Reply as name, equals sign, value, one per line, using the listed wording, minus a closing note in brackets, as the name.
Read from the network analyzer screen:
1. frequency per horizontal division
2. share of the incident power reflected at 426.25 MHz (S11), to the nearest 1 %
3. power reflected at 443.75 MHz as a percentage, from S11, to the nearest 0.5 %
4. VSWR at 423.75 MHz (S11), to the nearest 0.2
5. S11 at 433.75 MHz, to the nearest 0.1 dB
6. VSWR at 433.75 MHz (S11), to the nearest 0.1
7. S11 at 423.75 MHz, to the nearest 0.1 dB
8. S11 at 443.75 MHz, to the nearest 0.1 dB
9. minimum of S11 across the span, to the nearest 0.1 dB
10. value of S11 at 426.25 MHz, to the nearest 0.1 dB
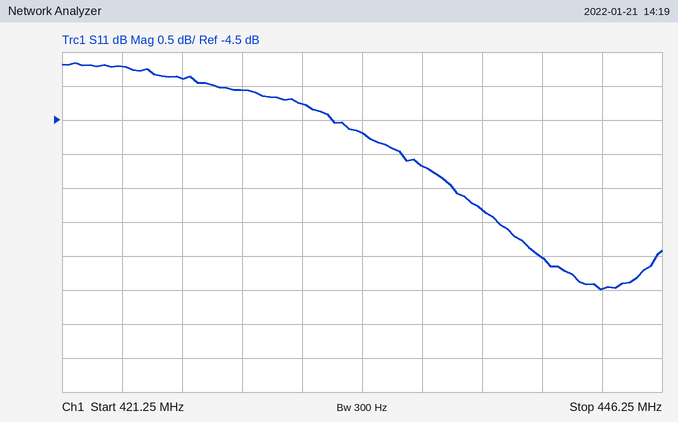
frequency per horizontal division = 2.5 MHz
share of the incident power reflected at 426.25 MHz (S11), to the nearest 1 % = 41 %
power reflected at 443.75 MHz as a percentage, from S11, to the nearest 0.5 % = 20.0 %
VSWR at 423.75 MHz (S11), to the nearest 0.2 = 4.8
S11 at 433.75 MHz, to the nearest 0.1 dB = -4.7 dB
VSWR at 433.75 MHz (S11), to the nearest 0.1 = 3.8
S11 at 423.75 MHz, to the nearest 0.1 dB = -3.7 dB
S11 at 443.75 MHz, to the nearest 0.1 dB = -7.0 dB
minimum of S11 across the span, to the nearest 0.1 dB = -7.0 dB
value of S11 at 426.25 MHz, to the nearest 0.1 dB = -3.9 dB
